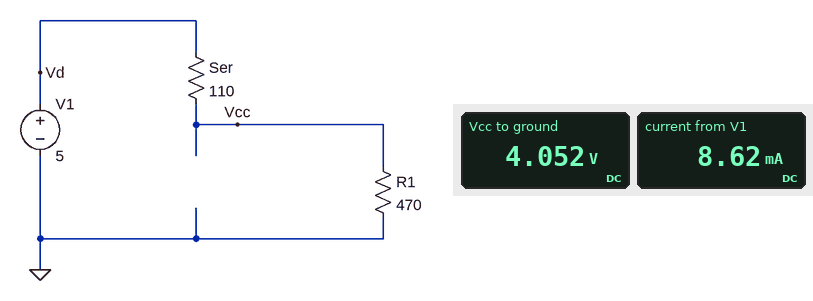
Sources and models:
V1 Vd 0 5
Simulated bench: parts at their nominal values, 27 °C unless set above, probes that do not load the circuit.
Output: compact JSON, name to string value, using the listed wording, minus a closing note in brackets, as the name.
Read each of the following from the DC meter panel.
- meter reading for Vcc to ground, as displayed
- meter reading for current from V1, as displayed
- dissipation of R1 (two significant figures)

{"meter reading for Vcc to ground, as displayed": "4.052 V", "meter reading for current from V1, as displayed": "8.62 mA", "dissipation of R1": "35 mW"}
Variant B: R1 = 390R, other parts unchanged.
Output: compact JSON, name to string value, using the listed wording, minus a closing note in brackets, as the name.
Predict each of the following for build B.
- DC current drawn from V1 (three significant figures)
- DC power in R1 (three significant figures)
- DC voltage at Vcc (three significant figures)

{"DC current drawn from V1": "10.0 mA", "DC power in R1": "39.0 mW", "DC voltage at Vcc": "3.90 V"}
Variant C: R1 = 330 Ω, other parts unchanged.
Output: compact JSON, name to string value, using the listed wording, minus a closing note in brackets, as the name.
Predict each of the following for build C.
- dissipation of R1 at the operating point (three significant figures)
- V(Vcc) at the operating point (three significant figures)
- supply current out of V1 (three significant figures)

{"dissipation of R1 at the operating point": "42.6 mW", "V(Vcc) at the operating point": "3.75 V", "supply current out of V1": "11.4 mA"}
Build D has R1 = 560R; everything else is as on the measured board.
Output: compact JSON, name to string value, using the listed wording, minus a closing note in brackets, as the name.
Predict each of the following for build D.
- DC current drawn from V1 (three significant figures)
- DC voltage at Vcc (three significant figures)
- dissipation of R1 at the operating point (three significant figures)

{"DC current drawn from V1": "7.46 mA", "DC voltage at Vcc": "4.18 V", "dissipation of R1 at the operating point": "31.2 mW"}
